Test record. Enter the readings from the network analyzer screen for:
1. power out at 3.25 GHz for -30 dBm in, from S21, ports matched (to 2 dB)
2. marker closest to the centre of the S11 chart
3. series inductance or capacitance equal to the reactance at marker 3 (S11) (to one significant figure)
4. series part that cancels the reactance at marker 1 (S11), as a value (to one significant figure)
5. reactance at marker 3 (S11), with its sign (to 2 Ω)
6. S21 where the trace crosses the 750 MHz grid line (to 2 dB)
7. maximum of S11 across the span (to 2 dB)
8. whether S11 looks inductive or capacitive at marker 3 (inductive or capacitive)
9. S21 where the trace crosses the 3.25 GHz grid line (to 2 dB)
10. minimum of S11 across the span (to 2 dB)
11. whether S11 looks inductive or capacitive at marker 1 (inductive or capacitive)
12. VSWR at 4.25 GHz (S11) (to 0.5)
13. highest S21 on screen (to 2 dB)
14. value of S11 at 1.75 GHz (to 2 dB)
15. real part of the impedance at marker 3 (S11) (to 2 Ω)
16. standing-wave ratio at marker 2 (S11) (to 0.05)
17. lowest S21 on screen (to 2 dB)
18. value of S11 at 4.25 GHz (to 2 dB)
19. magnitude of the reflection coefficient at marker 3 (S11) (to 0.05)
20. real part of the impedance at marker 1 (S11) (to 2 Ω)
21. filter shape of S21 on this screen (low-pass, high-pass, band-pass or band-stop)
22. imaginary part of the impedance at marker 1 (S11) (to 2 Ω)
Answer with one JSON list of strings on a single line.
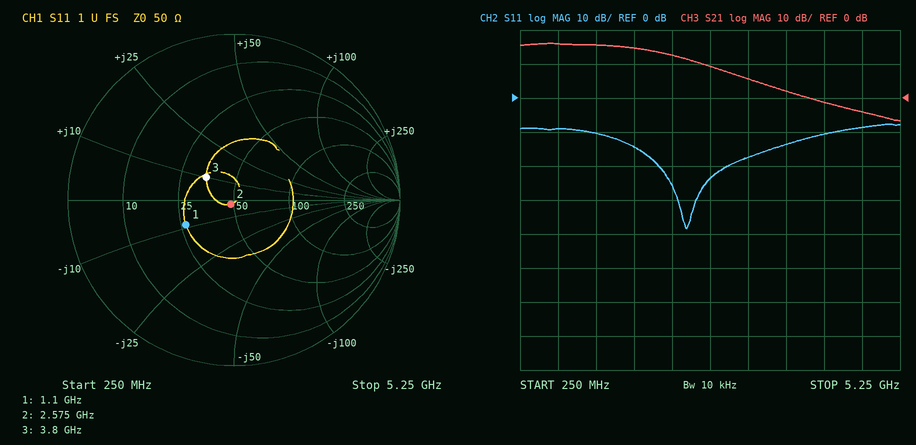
["-24 dBm", "marker 2", "400 pH", "1 nH", "+10 Ω", "16 dB", "-8 dB", "inductive", "6 dB", "-38 dB", "capacitive", "2.0", "16 dB", "-14 dB", "34 Ω", "1.05", "-6 dB", "-10 dB", "0.20", "26 Ω", "low-pass", "-8 Ω"]
